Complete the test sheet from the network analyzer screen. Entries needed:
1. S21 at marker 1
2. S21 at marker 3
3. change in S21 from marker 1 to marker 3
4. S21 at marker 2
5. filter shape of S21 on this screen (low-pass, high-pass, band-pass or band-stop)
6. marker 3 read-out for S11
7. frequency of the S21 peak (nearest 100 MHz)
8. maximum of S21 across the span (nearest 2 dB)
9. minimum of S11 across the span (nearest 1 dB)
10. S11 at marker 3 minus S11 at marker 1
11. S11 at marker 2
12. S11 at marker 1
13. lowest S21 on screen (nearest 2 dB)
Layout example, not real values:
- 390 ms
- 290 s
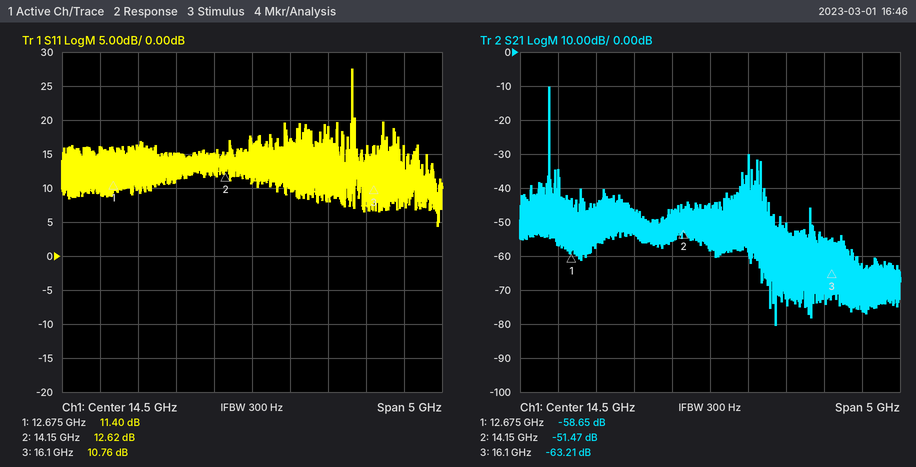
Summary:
- -58.65 dB
- -63.21 dB
- -4.56 dB
- -51.47 dB
- band-pass
- 10.76 dB
- 12.4 GHz
- -10 dB
- 4 dB
- -0.64 dB
- 12.62 dB
- 11.40 dB
- -80 dB
